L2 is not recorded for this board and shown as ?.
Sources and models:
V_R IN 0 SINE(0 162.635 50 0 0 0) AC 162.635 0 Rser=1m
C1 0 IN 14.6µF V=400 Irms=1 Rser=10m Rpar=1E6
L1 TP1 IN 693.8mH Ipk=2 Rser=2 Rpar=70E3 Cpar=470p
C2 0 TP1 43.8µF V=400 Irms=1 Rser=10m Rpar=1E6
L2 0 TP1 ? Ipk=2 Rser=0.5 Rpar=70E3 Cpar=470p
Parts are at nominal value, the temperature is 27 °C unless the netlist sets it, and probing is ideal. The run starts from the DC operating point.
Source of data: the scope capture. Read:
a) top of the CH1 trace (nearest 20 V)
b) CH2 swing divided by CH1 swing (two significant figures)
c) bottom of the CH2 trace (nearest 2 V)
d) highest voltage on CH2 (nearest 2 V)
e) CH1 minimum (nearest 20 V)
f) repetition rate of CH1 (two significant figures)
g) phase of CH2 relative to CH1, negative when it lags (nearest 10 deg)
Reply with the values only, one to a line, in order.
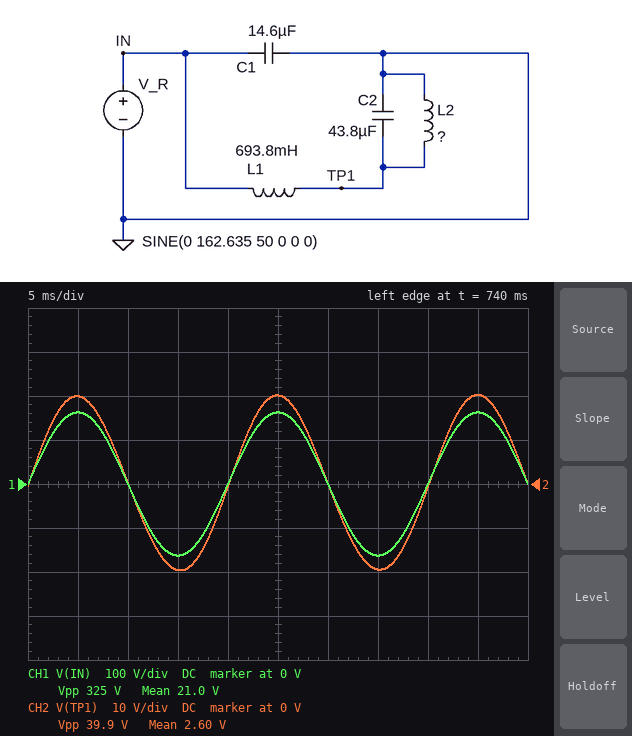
160 V
0.12
-20 V
20 V
-160 V
50 Hz
0 deg
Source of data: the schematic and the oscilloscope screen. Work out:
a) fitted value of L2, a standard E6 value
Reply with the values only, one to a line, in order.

68 mH
